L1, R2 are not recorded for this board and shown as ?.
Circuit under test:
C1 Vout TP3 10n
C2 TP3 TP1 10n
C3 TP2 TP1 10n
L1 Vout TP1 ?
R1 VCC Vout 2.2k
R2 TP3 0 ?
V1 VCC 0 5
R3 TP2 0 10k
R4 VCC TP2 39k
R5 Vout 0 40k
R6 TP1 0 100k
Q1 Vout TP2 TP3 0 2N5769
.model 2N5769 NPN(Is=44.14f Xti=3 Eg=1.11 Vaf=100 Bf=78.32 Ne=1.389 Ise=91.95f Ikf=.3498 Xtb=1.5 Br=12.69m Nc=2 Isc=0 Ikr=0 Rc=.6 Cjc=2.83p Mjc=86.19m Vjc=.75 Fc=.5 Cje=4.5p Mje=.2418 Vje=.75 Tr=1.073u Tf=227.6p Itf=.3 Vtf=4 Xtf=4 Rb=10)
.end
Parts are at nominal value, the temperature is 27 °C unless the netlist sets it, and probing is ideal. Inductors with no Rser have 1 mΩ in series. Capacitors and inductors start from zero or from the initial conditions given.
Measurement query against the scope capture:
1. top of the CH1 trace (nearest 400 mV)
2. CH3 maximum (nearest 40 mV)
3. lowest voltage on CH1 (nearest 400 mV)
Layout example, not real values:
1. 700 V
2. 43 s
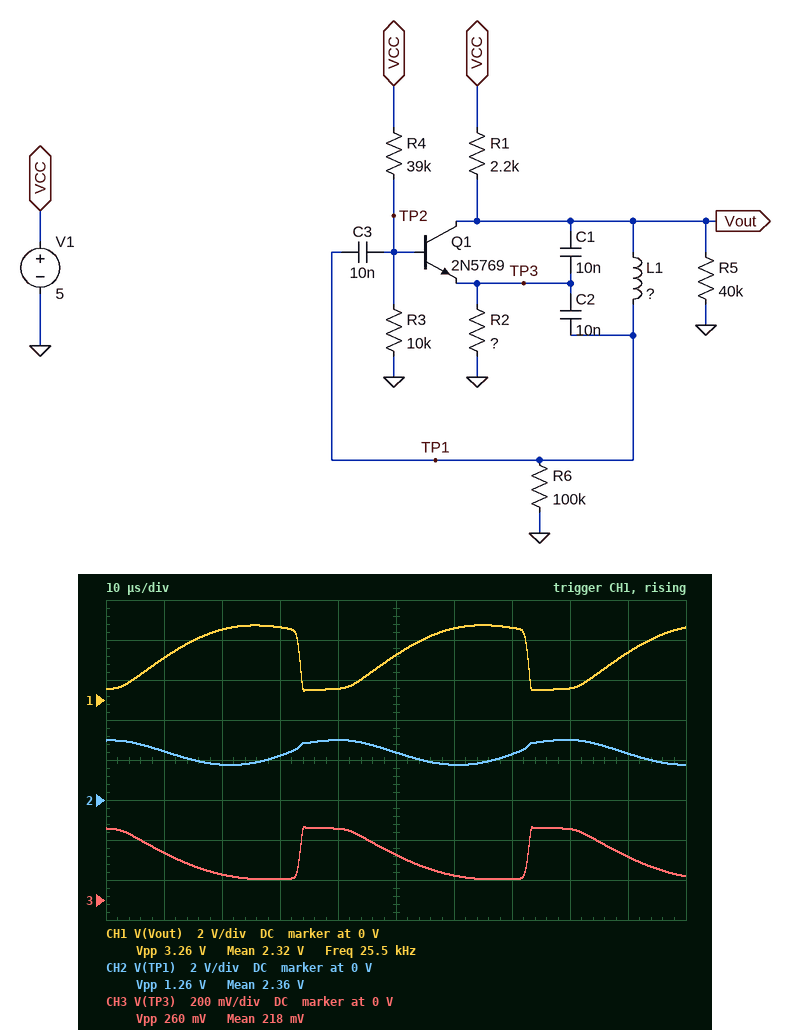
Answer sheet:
1. 3.6 V
2. 360 mV
3. 400 mV
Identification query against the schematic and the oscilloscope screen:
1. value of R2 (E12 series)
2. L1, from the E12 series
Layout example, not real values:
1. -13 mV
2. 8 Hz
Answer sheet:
1. 180 Ω
2. 15 mH
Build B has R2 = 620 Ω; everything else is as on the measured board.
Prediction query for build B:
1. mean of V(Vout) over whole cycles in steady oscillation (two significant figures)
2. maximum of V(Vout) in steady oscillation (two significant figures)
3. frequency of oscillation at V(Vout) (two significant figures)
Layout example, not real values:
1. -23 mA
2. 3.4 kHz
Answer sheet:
1. 2.9 V
2. 4.1 V
3. 23 kHz
